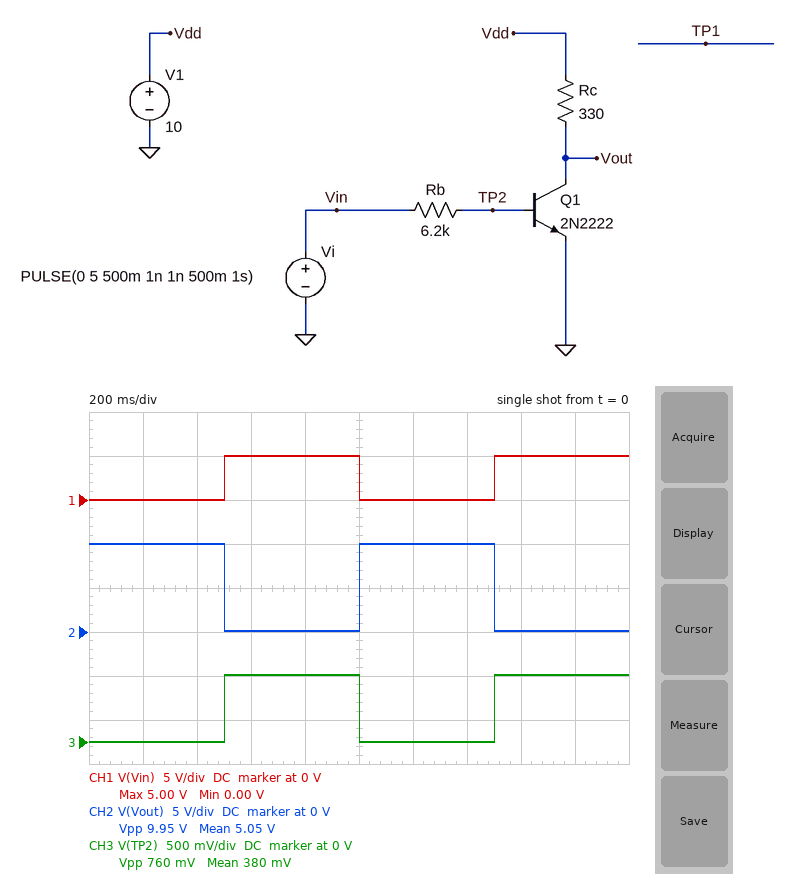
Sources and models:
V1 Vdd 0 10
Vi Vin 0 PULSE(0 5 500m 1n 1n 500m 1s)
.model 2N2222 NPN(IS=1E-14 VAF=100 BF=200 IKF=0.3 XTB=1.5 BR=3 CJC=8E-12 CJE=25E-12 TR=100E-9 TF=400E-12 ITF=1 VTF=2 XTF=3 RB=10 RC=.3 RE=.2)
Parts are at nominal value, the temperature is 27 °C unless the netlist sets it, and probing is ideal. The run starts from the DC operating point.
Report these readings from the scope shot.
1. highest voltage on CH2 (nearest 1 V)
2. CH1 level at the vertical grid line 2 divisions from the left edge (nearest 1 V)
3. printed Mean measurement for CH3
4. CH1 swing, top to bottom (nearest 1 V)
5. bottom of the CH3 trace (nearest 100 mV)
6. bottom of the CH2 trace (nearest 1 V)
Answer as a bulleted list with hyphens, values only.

- 10 V
- 0 V
- 380 mV
- 5 V
- 0 V
- 0 V
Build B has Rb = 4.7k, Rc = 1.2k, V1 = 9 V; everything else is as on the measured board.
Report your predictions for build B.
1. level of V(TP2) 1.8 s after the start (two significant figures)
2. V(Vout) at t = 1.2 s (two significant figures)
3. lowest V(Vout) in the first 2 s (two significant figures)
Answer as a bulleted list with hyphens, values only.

- 730 mV
- 9.0 V
- 39 mV
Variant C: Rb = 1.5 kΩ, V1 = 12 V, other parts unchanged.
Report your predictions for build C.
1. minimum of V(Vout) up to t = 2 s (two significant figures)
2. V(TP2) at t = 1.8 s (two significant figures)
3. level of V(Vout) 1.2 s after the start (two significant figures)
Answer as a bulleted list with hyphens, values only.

- 66 mV
- 790 mV
- 12 V
